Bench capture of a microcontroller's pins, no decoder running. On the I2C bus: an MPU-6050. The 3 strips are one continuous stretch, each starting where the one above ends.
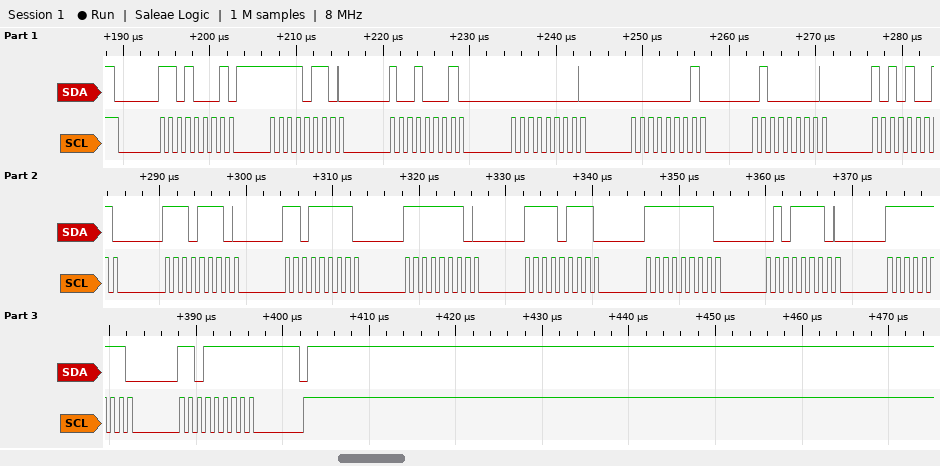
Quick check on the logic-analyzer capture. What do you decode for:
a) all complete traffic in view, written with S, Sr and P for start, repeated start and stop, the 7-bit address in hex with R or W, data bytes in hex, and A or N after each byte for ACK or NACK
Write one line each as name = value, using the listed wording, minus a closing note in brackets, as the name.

all complete traffic in view, written with S, Sr and P for start, repeated start and stop, the 7-bit address in hex with R or W, data bytes in hex, and A or N after each byte for ACK or NACK = S 68R A F6 A 91 A 00 A 01 A 40 A A9 A EE A DF A FE A F7 A FF A 5E A FF A DF N P
